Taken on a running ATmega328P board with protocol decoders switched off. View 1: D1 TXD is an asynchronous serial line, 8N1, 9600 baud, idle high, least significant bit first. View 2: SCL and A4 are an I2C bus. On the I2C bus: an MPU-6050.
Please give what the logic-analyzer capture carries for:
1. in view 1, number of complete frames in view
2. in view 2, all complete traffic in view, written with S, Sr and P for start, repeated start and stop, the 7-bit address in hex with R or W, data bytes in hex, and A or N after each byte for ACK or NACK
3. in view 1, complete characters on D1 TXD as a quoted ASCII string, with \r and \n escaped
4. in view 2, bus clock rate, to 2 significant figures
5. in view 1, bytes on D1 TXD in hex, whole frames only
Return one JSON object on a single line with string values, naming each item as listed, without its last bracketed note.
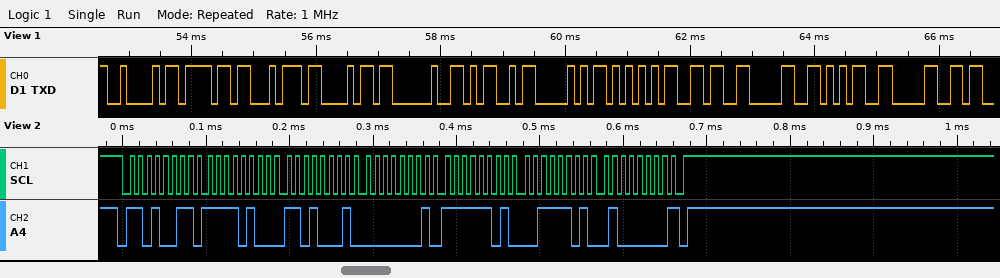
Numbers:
{"in view 1, number of complete frames in view": "12", "in view 2, all complete traffic in view, written with S, Sr and P for start, repeated start and stop, the 7-bit address in hex with R or W, data bytes in hex, and A or N after each byte for ACK or NACK": "S 69R A F4 A D1 A 01 A FD A 3D A 40 N P", "in view 1, complete characters on D1 TXD as a quoted ASCII string, with \\r and \\n escaped": "\"Both MPU6050\"", "in view 2, bus clock rate, to 2 significant figures": "100 kHz", "in view 1, bytes on D1 TXD in hex, whole frames only": "42 6F 74 68 20 4D 50 55 36 30 35 30"}
